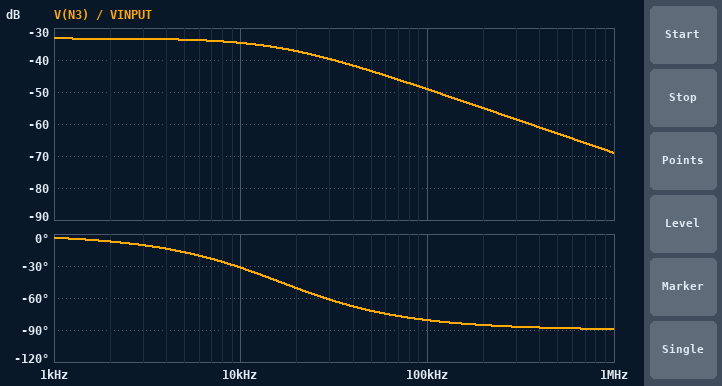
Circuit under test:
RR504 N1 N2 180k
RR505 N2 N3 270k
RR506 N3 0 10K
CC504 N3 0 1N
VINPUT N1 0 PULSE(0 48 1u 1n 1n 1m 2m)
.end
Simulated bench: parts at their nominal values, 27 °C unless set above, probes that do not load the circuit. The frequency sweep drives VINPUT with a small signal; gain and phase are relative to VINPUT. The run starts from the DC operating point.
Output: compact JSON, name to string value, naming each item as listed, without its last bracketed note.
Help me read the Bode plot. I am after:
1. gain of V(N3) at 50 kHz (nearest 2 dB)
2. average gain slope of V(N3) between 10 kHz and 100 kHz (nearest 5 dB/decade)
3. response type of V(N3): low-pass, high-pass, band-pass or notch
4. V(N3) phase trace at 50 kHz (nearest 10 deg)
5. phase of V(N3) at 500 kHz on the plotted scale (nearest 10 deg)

{"gain of V(N3) at 50 kHz": "-44 dB", "average gain slope of V(N3) between 10 kHz and 100 kHz": "-15 dB/decade", "response type of V(N3): low-pass, high-pass, band-pass or notch": "low-pass", "V(N3) phase trace at 50 kHz": "-70 deg", "phase of V(N3) at 500 kHz on the plotted scale": "-90 deg"}
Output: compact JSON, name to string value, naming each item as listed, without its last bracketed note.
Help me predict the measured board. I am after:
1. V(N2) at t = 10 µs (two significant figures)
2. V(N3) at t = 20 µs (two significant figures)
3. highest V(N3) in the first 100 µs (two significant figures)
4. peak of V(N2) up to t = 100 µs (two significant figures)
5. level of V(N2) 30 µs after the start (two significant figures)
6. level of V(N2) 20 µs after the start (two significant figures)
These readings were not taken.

{"V(N2) at t = 10 µs": "29 V", "V(N3) at t = 20 µs": "890 mV", "highest V(N3) in the first 100 µs": "1.0 V", "peak of V(N2) up to t = 100 µs": "29 V", "level of V(N2) 30 µs after the start": "29 V", "level of V(N2) 20 µs after the start": "29 V"}
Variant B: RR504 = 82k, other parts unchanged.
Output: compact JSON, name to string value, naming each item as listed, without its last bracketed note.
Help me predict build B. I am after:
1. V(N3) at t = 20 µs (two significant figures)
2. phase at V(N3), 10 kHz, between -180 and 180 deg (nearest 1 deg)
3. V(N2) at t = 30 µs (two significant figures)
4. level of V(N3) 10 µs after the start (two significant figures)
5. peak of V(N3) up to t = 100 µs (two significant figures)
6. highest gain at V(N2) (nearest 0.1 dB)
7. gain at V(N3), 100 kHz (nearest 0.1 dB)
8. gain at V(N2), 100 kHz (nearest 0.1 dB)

{"V(N3) at t = 20 µs": "1.1 V", "phase at V(N3), 10 kHz, between -180 and 180 deg": "-31 deg", "V(N2) at t = 30 µs": "37 V", "level of V(N3) 10 µs after the start": "800 mV", "peak of V(N3) up to t = 100 µs": "1.3 V", "highest gain at V(N2)": "-2.2 dB", "gain at V(N3), 100 kHz": "-47.0 dB", "gain at V(N2), 100 kHz": "-2.3 dB"}
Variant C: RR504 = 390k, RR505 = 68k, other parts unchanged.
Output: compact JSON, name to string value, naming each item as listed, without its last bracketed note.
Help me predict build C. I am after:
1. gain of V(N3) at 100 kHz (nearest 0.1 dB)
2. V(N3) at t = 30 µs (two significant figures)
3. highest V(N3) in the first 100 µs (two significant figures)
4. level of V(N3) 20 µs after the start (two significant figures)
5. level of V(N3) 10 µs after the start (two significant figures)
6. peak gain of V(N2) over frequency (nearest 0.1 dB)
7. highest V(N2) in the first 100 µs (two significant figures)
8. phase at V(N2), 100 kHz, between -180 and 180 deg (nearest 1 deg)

{"gain of V(N3) at 100 kHz": "-49.3 dB", "V(N3) at t = 30 µs": "970 mV", "highest V(N3) in the first 100 µs": "1.0 V", "level of V(N3) 20 µs after the start": "880 mV", "level of V(N3) 10 µs after the start": "620 mV", "peak gain of V(N2) over frequency": "-15.6 dB", "highest V(N2) in the first 100 µs": "8.0 V", "phase at V(N2), 100 kHz, between -180 and 180 deg": "-1 deg"}
